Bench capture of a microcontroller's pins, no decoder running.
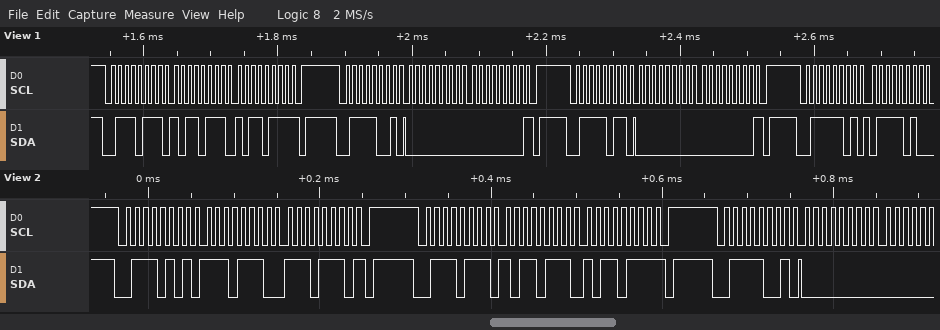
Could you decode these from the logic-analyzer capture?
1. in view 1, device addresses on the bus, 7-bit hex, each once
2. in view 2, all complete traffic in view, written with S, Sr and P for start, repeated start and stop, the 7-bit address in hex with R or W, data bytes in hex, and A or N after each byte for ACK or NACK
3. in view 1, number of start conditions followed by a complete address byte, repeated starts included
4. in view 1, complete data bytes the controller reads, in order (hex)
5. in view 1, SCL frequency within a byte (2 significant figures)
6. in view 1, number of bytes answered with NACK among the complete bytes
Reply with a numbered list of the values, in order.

1. 0x3B 0x3C 0x3D 0x3E
2. S 3AR A EE A EE N P S 3BR A B7 A B7 N P S 3CR A 00 A
3. 4
4. B7 B7 00 00 00 00 7A
5. 100 kHz
6. 3
